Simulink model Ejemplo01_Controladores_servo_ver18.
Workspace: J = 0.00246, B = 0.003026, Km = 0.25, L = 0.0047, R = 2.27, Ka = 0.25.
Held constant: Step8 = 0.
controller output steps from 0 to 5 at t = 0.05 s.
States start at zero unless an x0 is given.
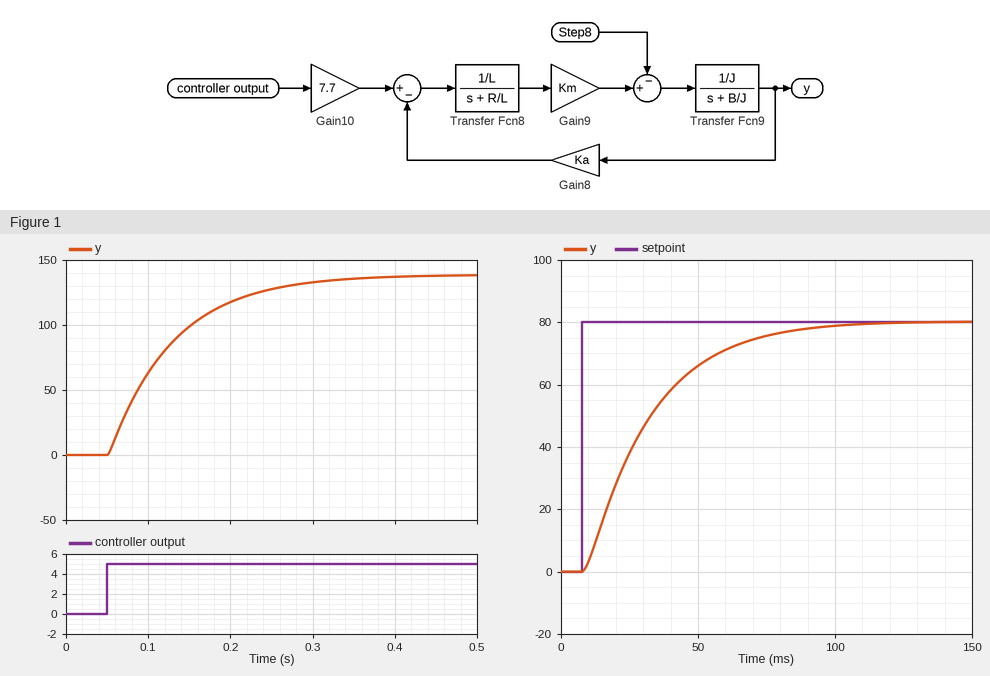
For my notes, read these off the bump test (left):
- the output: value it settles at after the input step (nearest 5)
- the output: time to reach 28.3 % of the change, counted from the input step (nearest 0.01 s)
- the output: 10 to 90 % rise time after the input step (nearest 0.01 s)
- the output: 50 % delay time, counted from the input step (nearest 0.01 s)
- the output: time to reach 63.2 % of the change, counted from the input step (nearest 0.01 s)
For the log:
140
0.03 s
0.17 s
0.06 s
0.08 s
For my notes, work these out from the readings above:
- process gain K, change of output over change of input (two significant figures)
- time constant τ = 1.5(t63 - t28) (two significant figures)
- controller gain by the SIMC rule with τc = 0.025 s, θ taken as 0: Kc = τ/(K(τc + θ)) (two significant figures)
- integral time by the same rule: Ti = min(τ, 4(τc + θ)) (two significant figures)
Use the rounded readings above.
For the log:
28
0.075 s
0.11
0.075 s
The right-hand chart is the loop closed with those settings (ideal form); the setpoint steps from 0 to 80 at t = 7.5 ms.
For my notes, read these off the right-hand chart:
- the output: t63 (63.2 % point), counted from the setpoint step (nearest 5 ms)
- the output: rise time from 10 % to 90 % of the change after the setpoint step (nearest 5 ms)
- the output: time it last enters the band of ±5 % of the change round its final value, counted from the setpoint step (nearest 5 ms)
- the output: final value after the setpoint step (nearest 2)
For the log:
25 ms
50 ms
70 ms
80
